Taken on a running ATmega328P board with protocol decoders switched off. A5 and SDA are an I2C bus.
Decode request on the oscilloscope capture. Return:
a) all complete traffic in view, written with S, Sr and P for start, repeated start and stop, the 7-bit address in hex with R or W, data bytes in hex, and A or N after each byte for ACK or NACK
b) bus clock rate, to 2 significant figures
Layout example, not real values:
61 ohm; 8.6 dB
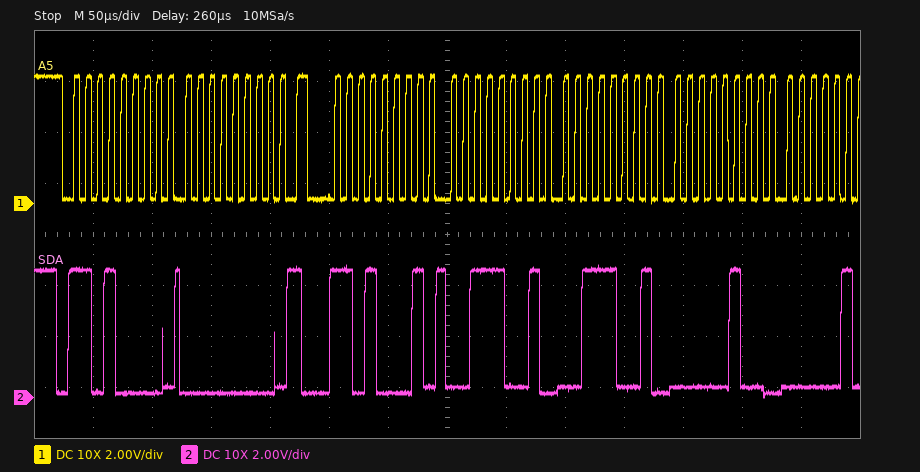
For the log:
S 68W A 00 A Sr 68R A 39 A 39 A 04 A; 100 kHz
